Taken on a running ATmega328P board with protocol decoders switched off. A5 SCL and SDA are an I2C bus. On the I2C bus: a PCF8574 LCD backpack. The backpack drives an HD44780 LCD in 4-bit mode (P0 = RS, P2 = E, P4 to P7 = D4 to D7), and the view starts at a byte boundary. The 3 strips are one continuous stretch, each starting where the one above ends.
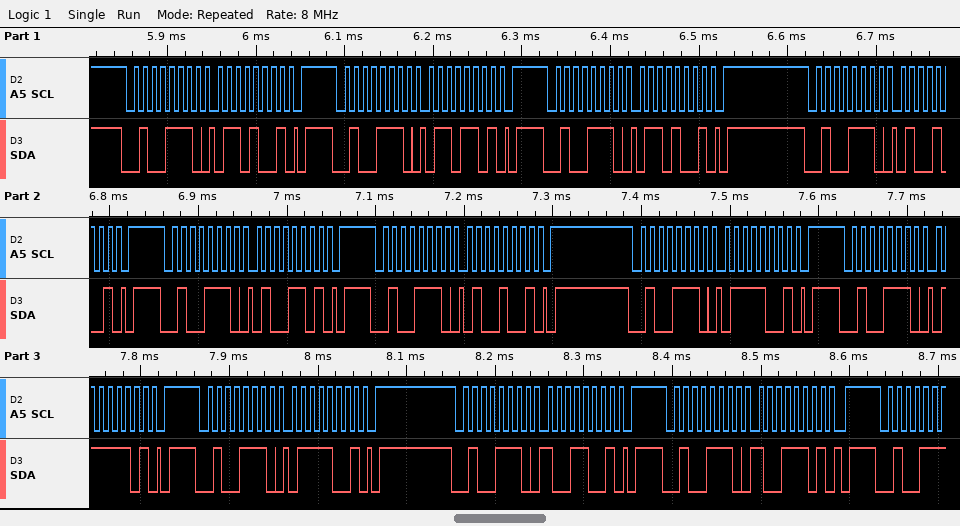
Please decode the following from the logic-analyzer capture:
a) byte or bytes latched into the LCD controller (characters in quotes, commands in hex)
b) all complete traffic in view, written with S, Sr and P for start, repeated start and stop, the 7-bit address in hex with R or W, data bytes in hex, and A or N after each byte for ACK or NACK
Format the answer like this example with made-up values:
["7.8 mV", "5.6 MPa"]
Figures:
["'d'", "S 27W A 69 A P S 27W A 6D A P S 27W A 69 A P S 27W A 49 A P S 27W A 4D A P S 27W A 49 A P S 27W A 79 A P S 27W A 7D A P S 27W A 79 A P S 27W A 99 A P S 27W A 9D A P"]
